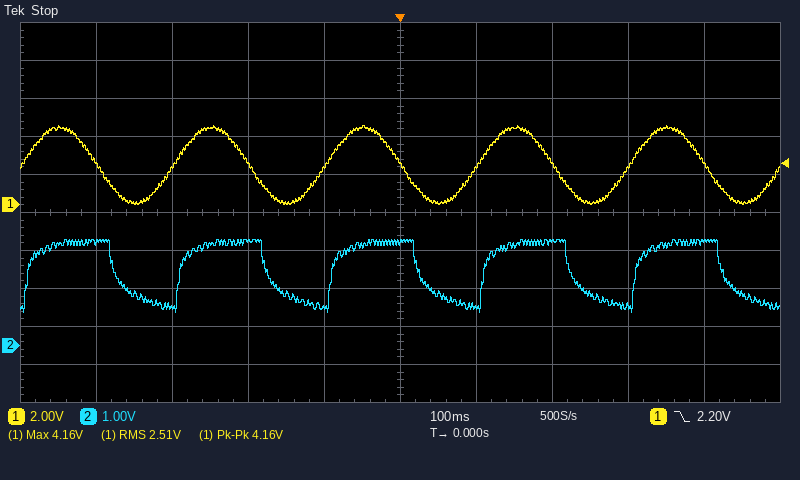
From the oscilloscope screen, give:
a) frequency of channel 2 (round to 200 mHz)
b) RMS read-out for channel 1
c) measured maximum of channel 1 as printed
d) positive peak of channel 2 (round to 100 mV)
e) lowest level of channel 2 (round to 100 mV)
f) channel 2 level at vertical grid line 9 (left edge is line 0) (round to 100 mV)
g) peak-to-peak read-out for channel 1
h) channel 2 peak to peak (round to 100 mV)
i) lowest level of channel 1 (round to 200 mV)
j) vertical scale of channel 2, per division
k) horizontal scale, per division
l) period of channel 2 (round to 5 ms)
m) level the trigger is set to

5.0 Hz
2.51 V
4.16 V
2.8 V
900 mV
2.7 V
4.16 V
1.9 V
0.0 V
1 V
100 ms
200 ms
2.20 V
